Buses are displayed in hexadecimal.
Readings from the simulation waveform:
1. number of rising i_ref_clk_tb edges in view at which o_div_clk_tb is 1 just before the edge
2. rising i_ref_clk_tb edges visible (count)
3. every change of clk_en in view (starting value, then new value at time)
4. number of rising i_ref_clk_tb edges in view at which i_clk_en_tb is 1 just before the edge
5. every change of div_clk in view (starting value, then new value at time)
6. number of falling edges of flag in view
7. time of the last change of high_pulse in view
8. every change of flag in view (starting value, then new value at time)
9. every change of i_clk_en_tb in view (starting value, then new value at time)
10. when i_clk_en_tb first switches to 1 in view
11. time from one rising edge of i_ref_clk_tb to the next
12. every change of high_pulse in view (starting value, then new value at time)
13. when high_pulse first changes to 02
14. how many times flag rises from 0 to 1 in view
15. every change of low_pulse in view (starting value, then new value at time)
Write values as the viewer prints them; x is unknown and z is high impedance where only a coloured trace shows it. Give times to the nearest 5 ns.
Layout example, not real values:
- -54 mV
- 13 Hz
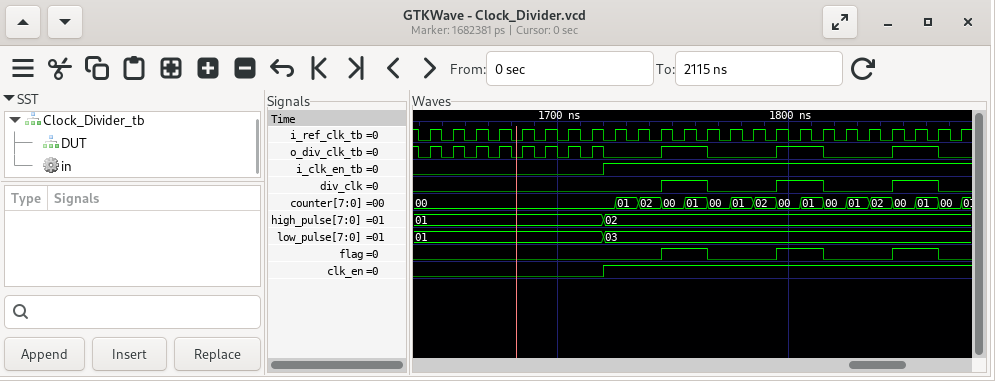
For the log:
- 6
- 24
- 0, 1 at 1720 ns
- 16
- 0, 1 at 1745 ns, 0 at 1765 ns, 1 at 1795 ns, 0 at 1815 ns, 1 at 1845 ns, 0 at 1865 ns
- 3
- 1720 ns
- 0, 1 at 1745 ns, 0 at 1765 ns, 1 at 1795 ns, 0 at 1815 ns, 1 at 1845 ns, 0 at 1865 ns
- 0, 1 at 1720 ns
- 1720 ns
- 10 ns
- 01, 02 at 1720 ns
- 1720 ns
- 3
- 01, 03 at 1720 ns
